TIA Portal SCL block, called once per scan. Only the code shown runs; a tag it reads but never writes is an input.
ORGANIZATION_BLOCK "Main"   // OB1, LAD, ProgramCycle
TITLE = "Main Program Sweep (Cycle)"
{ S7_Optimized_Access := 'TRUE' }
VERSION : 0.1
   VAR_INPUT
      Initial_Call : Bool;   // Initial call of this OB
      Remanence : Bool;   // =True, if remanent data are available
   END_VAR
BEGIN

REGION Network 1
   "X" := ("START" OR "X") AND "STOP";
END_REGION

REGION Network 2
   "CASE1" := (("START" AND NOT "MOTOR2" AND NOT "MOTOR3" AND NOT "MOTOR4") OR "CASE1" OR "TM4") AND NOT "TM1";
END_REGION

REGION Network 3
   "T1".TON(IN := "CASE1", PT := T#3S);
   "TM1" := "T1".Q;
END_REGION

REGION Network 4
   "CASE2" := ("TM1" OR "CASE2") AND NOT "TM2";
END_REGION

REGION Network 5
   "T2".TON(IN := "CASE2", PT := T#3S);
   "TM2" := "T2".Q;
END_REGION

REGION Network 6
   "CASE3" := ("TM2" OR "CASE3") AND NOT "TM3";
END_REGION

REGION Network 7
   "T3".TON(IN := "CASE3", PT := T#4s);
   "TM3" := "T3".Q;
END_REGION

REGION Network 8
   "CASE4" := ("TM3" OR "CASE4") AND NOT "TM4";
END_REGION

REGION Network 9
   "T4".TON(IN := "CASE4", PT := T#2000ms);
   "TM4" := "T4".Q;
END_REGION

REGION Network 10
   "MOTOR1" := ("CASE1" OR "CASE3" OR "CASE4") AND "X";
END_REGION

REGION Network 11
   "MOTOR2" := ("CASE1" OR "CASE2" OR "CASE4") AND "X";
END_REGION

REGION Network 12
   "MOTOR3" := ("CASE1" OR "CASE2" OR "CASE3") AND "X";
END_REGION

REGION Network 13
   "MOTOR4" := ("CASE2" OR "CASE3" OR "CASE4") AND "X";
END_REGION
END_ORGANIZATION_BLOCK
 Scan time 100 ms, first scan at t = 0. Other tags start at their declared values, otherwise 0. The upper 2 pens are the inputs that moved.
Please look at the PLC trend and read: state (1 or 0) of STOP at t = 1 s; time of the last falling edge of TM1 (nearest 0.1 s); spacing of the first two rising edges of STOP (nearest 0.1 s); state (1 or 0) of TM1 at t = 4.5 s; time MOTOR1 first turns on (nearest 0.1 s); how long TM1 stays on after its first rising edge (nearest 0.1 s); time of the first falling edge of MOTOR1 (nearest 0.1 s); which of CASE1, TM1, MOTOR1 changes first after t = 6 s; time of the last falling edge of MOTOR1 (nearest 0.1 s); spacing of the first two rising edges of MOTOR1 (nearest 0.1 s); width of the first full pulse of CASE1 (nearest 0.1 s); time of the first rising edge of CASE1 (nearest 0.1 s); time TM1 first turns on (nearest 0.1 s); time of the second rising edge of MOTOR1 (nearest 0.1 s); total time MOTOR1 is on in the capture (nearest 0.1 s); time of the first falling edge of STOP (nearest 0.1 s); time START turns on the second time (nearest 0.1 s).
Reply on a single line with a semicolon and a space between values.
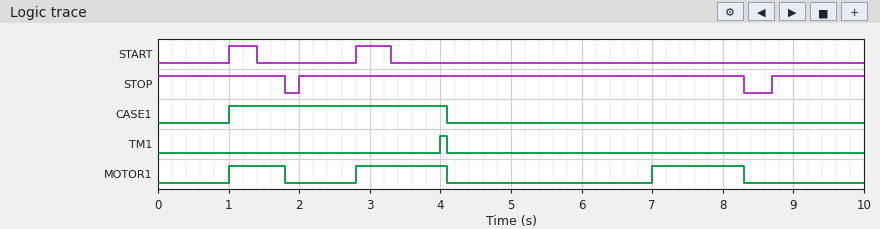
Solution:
1; 4.1 s; 6.7 s; 0; 1.0 s; 0.1 s; 1.8 s; MOTOR1; 8.3 s; 1.8 s; 3.1 s; 1.0 s; 4.0 s; 2.8 s; 3.4 s; 1.8 s; 2.8 s
